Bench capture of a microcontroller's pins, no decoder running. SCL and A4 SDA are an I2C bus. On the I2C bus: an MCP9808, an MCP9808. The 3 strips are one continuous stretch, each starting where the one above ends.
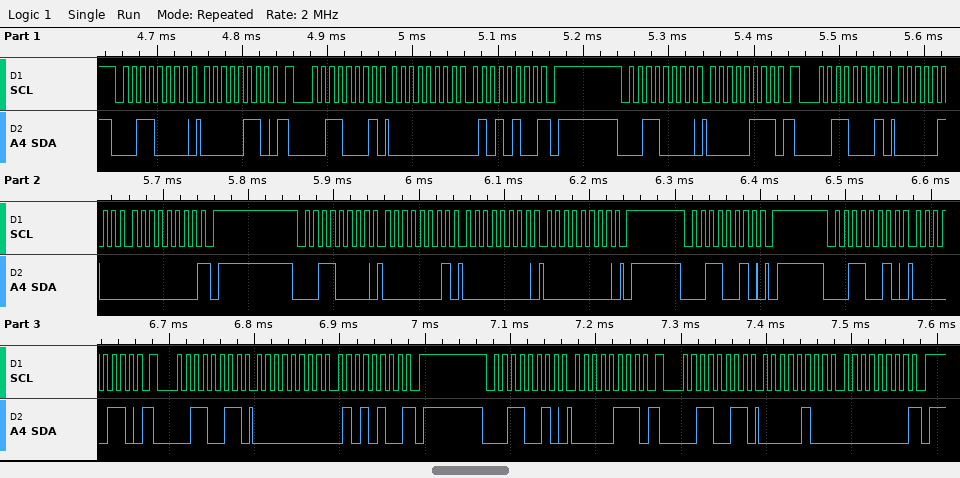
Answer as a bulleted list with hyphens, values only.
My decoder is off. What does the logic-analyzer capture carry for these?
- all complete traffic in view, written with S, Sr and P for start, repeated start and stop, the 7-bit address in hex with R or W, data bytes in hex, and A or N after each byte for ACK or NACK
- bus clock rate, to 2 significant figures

- S 18W A 06 A Sr 18R A 00 A 54 N P S 18W A 07 A Sr 18R A 04 A 00 N P S 18W A 01 A 00 A 00 A P S 19W A P S 19W A 06 A Sr 19R A 00 A 54 N P S 19W A 07 A Sr 19R A 04 A 00 N P
- 100 kHz
